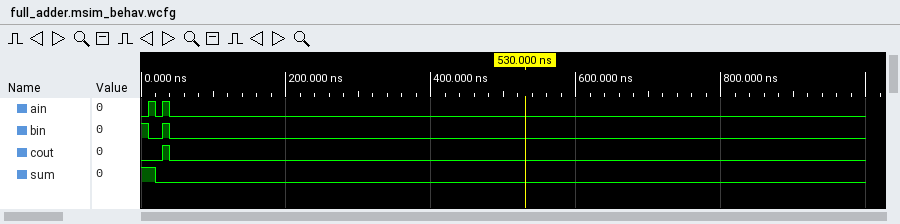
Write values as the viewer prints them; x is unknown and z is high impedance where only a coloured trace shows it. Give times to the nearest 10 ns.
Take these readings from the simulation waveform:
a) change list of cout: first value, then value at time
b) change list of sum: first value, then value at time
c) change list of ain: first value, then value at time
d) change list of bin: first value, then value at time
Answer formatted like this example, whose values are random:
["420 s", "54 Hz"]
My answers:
["0, 1 at 30 ns, 0 at 40 ns", "1, 0 at 20 ns", "0, 1 at 10 ns, 0 at 20 ns, 1 at 30 ns, 0 at 40 ns", "1, 0 at 10 ns, 1 at 30 ns, 0 at 40 ns"]
